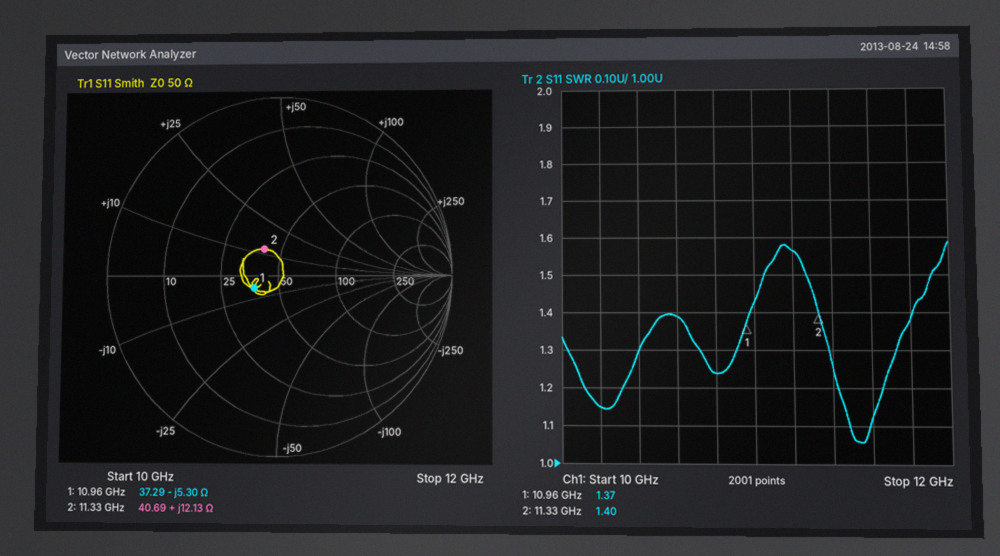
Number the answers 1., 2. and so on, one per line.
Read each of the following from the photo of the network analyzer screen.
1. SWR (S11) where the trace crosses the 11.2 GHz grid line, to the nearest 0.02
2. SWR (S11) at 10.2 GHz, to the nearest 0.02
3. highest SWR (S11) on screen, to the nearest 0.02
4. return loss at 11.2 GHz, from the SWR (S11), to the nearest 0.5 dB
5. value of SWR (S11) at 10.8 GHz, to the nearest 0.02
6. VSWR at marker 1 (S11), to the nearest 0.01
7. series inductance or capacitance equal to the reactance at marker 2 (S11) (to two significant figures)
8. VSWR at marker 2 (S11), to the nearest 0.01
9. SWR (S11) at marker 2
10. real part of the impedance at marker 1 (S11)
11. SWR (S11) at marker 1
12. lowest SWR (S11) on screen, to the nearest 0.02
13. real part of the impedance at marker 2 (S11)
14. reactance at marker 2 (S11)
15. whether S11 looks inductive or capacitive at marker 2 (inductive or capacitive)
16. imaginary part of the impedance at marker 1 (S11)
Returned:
1. 1.56
2. 1.14
3. 1.58
4. 13.0 dB
5. 1.24
6. 1.37
7. 170 pH
8. 1.40
9. 1.40
10. 37.29 Ω
11. 1.37
12. 1.06
13. 40.69 Ω
14. +12.13 Ω
15. inductive
16. -5.30 Ω
